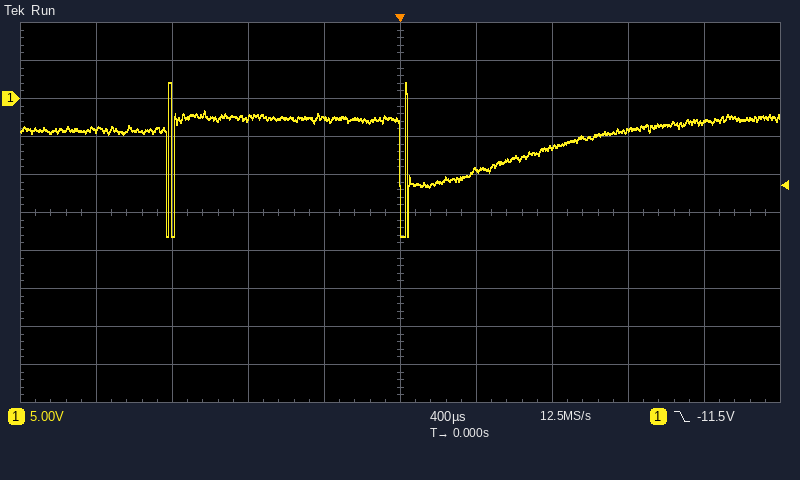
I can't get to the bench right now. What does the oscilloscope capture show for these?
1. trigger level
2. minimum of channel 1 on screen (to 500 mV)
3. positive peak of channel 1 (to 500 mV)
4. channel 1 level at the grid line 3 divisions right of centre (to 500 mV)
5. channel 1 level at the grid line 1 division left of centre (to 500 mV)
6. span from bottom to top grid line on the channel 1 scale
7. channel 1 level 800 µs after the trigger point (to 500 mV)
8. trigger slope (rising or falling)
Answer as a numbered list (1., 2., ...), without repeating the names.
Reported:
1. -11.5 V
2. -18.0 V
3. 2.0 V
4. -4.0 V
5. -2.5 V
6. 50 V
7. -6.5 V
8. falling
